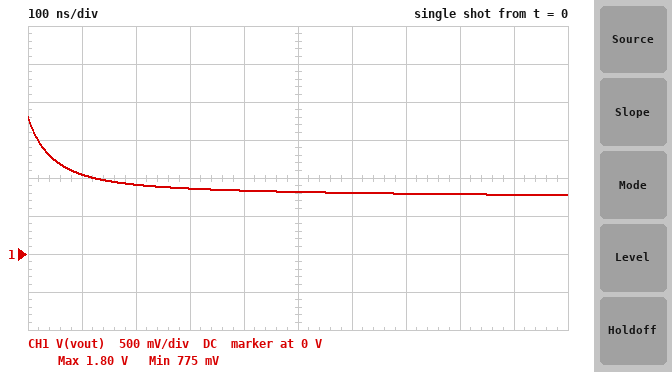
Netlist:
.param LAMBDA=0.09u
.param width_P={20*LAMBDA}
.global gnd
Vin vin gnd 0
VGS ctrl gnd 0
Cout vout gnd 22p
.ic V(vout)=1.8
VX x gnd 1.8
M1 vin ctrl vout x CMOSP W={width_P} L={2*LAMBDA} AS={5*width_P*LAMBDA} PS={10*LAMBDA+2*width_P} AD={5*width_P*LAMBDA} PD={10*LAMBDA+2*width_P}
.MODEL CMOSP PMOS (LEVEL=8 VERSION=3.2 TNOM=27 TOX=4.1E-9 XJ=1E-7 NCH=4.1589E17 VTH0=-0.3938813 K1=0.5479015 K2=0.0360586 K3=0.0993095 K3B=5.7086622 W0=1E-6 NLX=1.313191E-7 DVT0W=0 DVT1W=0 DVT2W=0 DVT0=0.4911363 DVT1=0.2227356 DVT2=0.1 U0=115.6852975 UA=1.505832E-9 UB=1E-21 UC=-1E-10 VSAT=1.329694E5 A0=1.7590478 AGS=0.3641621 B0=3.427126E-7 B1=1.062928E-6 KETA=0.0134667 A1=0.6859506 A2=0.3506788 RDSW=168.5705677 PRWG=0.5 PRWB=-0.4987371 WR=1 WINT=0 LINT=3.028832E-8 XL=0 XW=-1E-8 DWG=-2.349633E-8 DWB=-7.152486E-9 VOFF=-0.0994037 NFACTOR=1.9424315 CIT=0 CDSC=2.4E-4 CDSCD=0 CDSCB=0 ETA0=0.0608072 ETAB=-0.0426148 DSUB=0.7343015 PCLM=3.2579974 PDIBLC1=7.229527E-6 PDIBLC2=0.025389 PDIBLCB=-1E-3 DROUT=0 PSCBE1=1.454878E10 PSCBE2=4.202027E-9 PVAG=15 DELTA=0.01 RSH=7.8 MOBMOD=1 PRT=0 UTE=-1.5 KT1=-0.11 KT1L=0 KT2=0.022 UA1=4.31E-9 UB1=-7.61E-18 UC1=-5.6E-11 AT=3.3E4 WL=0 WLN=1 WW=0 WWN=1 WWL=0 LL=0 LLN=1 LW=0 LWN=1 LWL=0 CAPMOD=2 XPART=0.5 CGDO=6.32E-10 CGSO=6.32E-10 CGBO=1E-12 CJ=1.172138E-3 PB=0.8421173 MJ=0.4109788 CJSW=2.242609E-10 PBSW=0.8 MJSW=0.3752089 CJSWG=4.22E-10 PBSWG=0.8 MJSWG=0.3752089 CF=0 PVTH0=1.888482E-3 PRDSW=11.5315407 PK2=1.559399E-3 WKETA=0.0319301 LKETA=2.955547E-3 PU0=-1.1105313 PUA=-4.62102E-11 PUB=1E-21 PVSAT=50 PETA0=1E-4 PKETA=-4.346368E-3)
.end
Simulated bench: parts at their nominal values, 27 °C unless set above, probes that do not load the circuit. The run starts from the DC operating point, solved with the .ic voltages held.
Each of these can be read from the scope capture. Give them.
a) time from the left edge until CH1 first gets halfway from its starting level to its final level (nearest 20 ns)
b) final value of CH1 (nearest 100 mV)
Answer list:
40 ns
800 mV
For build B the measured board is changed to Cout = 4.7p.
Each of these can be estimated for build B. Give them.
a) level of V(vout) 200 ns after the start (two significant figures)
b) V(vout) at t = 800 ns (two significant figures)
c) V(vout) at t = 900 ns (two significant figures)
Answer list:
780 mV
720 mV
710 mV
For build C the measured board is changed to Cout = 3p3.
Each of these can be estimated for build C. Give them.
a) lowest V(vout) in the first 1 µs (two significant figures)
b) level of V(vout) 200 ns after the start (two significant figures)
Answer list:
700 mV
760 mV
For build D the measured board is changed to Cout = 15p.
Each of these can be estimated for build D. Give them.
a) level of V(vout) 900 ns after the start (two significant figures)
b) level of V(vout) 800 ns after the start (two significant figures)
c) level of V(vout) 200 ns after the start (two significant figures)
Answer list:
760 mV
770 mV
860 mV
